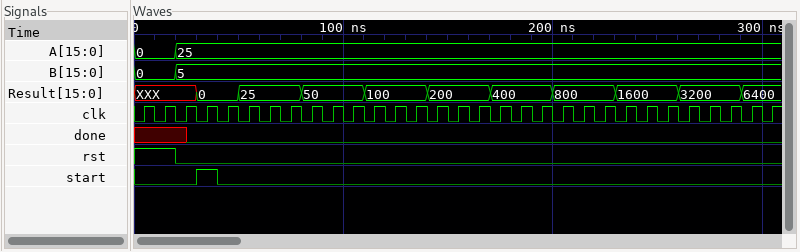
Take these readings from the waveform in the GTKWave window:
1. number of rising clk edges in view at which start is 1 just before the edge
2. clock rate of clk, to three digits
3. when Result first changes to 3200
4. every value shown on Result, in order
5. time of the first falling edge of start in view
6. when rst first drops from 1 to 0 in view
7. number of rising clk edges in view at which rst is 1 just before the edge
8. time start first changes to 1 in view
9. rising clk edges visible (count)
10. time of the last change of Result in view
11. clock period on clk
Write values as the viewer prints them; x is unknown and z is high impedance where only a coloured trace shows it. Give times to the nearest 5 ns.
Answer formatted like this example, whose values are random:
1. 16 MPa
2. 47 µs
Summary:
1. 1
2. 100 MHz
3. 260 ns
4. XXX, 0, 25, 50, 100, 200, 400, 800, 1600, 3200, 6400
5. 40 ns
6. 20 ns
7. 2
8. 30 ns
9. 31
10. 290 ns
11. 10 ns
